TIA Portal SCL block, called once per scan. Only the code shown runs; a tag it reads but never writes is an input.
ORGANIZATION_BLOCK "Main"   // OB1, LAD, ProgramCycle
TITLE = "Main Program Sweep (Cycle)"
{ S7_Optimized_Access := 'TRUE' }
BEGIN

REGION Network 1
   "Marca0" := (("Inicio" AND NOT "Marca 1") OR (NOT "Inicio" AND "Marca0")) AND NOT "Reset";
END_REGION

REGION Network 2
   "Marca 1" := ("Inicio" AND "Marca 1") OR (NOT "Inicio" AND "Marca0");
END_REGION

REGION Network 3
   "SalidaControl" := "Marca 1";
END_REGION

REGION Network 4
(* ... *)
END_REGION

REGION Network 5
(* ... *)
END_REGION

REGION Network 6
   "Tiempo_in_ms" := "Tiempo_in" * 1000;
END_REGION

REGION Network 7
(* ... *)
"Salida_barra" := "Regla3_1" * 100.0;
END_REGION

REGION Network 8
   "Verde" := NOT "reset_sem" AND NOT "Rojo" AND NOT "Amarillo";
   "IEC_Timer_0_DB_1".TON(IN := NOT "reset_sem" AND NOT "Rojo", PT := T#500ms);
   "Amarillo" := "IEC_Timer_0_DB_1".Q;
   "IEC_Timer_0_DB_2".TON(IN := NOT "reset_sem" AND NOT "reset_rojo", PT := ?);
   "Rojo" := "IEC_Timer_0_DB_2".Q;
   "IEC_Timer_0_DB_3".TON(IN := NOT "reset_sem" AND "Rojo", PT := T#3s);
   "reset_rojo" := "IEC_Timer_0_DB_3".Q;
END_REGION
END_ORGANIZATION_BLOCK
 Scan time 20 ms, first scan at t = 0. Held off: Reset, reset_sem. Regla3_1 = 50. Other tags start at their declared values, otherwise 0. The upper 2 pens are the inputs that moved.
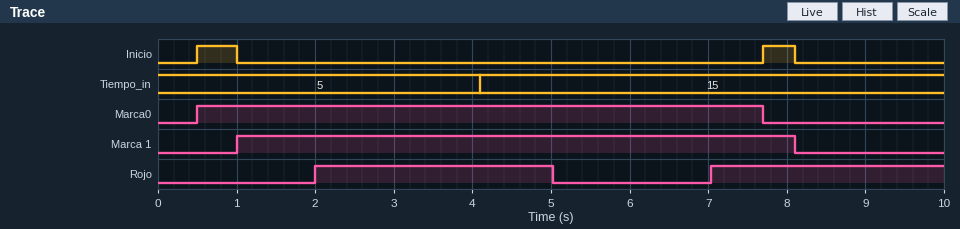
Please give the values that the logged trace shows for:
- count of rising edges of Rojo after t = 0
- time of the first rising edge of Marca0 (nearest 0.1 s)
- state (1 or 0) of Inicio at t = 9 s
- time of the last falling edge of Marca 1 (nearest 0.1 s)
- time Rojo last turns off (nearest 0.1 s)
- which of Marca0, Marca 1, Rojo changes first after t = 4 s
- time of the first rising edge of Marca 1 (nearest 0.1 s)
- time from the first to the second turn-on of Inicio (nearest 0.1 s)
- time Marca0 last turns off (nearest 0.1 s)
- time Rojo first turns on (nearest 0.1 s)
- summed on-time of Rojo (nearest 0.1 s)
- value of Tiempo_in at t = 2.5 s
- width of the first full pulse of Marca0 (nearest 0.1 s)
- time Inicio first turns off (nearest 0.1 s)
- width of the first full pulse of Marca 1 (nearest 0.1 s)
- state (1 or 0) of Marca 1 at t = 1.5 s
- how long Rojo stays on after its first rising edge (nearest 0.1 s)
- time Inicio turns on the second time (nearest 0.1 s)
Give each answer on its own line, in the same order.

2
0.5 s
0
8.1 s
5.0 s
Rojo
1.0 s
7.2 s
7.7 s
2.0 s
6.0 s
5
7.2 s
1.0 s
7.1 s
1
3.0 s
7.7 s
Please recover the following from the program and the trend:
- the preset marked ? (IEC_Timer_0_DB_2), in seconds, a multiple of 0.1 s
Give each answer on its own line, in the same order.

2.0 s
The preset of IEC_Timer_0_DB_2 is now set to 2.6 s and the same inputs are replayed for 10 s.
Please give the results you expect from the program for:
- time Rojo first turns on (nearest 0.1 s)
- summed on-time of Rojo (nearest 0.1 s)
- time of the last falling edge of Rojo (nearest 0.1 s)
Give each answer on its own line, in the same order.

2.6 s
4.8 s
5.6 s
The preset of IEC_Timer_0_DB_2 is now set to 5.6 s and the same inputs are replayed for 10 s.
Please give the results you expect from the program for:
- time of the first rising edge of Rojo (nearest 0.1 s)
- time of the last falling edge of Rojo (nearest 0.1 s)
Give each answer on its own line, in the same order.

5.6 s
8.6 s
